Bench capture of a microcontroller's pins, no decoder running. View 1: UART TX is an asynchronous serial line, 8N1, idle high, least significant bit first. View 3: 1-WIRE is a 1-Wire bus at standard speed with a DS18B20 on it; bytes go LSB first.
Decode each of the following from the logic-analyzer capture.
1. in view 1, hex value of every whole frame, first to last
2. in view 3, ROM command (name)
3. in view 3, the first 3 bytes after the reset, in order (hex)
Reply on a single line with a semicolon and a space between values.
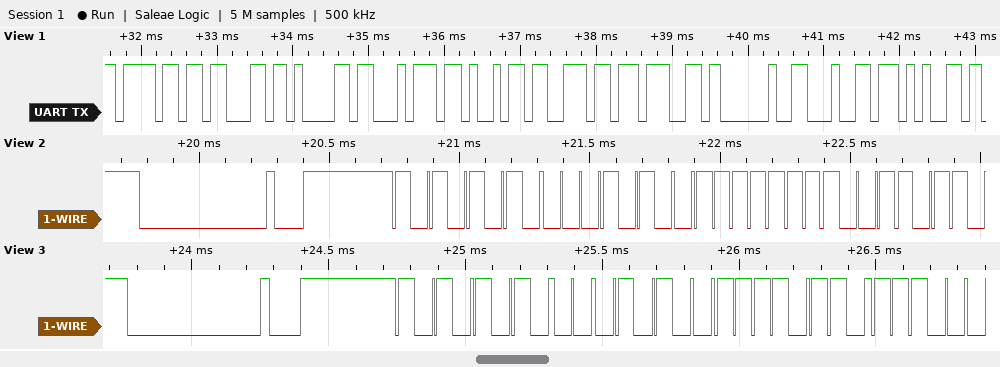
6F 63 61 74 69 6E 67 20 64 65; Match ROM; 55 28 6F
